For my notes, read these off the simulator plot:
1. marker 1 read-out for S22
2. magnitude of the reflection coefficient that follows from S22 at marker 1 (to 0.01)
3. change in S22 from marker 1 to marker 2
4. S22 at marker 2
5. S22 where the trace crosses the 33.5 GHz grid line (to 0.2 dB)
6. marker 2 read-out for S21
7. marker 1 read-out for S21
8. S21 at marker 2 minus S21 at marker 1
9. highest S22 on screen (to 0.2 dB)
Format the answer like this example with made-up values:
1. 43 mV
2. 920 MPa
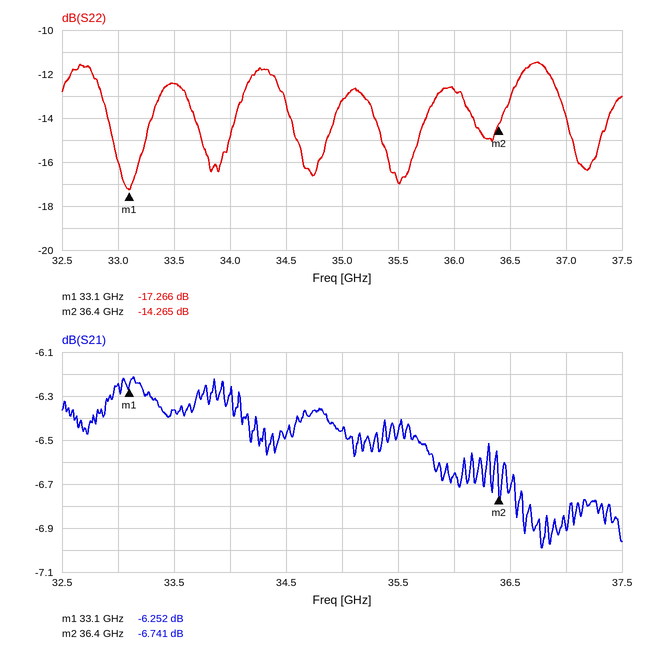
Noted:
1. -17.266 dB
2. 0.14
3. 3.001 dB
4. -14.265 dB
5. -12.4 dB
6. -6.741 dB
7. -6.252 dB
8. -0.489 dB
9. -11.4 dB
